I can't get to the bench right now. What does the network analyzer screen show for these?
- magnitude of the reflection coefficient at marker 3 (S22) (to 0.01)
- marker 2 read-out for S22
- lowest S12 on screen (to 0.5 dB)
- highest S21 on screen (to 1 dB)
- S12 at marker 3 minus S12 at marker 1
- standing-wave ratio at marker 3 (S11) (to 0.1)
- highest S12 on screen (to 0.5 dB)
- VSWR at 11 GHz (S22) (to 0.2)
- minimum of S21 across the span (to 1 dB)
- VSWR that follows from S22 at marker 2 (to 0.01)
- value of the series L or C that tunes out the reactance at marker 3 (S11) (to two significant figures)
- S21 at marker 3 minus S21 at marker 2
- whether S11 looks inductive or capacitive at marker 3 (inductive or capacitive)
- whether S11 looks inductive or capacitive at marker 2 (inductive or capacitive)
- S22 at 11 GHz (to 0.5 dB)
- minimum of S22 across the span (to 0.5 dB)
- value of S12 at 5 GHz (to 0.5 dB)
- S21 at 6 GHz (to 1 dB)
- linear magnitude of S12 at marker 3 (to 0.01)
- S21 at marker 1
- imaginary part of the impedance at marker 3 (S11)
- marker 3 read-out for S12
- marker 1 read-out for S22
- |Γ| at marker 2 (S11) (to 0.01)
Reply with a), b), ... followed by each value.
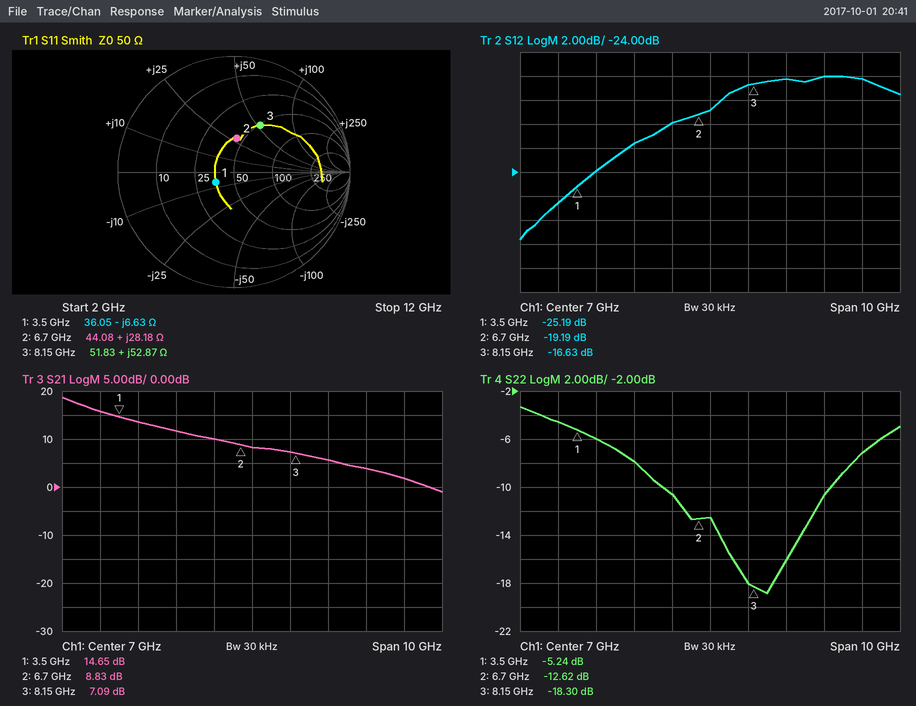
a) 0.12
b) -12.62 dB
c) -29.5 dB
d) 19 dB
e) 8.56 dB
f) 2.7
g) -16.0 dB
h) 2.6
i) -1 dB
j) 1.61
k) 370 fF
l) -1.74 dB
m) inductive
n) inductive
o) -7.0 dB
p) -19.0 dB
q) -21.5 dB
r) 10 dB
s) 0.15
t) 14.65 dB
u) +52.87 Ω
v) -16.63 dB
w) -5.24 dB
x) 0.29
